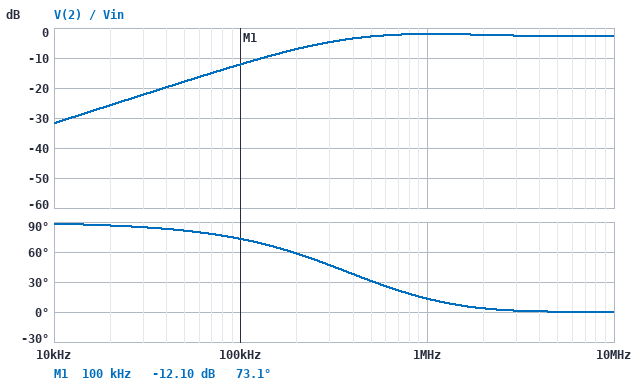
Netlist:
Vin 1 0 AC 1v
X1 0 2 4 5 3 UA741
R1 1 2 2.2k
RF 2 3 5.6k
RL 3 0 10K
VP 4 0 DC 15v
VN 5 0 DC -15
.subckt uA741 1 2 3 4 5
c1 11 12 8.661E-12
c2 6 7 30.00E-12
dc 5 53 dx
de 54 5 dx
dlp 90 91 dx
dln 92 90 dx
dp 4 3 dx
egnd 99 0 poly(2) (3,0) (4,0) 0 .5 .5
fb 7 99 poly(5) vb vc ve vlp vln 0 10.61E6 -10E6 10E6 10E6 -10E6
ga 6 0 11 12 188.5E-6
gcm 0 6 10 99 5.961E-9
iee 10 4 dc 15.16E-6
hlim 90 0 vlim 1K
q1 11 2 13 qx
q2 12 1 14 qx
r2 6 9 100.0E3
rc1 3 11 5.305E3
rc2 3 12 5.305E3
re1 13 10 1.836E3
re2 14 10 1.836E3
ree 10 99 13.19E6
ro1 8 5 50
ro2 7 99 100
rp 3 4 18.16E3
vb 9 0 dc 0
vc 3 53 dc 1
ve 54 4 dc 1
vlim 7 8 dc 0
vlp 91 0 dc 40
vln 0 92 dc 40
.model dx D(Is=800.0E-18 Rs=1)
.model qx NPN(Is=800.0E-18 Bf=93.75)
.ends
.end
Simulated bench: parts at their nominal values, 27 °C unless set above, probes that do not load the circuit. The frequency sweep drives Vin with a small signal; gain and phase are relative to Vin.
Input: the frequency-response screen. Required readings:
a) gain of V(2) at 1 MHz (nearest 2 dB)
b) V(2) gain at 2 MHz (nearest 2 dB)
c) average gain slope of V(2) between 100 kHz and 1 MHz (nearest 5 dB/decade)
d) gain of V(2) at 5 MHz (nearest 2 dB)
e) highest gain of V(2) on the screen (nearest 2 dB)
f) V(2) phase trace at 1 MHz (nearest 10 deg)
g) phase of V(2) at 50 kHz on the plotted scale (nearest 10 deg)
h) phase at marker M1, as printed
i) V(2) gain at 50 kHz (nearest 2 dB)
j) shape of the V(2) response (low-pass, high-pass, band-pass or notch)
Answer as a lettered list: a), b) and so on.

a) -2 dB
b) -2 dB
c) 10 dB/decade
d) -2 dB
e) -2 dB
f) 10 deg
g) 80 deg
h) 73.1 deg
i) -18 dB
j) high-pass
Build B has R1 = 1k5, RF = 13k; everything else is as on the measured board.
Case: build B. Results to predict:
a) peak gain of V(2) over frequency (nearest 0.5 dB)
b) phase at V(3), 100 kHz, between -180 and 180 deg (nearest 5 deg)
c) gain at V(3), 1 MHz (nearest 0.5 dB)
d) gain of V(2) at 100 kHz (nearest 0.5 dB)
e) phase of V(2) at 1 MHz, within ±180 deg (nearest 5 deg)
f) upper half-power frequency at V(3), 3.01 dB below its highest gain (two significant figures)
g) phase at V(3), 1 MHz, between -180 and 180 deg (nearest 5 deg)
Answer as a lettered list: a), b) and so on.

a) -0.5 dB
b) 135 deg
c) -2.0 dB
d) -4.0 dB
e) 5 deg
f) 110 kHz
g) 65 deg
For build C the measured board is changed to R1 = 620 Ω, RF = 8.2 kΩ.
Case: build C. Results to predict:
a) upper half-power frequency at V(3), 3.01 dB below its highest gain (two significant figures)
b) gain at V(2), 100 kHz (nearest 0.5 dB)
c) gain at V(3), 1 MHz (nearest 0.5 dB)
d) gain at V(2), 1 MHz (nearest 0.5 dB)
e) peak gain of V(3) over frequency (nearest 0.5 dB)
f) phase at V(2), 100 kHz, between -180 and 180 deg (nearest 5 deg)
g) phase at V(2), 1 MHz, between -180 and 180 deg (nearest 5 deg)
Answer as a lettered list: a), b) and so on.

a) 72 kHz
b) -2.0 dB
c) -1.5 dB
d) -0.5 dB
e) 22.5 dB
f) 35 deg
g) 5 deg
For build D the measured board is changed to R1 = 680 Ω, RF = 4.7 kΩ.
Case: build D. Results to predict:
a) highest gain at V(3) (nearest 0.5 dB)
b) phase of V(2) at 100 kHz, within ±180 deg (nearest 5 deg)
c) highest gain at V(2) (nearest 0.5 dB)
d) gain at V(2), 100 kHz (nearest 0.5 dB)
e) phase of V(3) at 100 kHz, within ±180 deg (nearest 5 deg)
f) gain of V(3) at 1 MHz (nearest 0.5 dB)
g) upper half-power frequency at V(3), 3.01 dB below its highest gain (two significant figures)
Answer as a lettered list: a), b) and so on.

a) 17.0 dB
b) 55 deg
c) -0.5 dB
d) -5.0 dB
e) 140 deg
f) -2.0 dB
g) 130 kHz
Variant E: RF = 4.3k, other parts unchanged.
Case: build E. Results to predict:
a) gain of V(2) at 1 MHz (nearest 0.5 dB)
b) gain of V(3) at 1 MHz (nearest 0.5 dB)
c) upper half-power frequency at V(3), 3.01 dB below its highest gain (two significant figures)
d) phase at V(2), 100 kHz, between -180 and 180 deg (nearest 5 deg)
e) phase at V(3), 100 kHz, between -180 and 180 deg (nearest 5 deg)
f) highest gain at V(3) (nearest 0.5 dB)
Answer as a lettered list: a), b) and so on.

a) -2.5 dB
b) -4.0 dB
c) 410 kHz
d) 75 deg
e) 165 deg
f) 6.0 dB
